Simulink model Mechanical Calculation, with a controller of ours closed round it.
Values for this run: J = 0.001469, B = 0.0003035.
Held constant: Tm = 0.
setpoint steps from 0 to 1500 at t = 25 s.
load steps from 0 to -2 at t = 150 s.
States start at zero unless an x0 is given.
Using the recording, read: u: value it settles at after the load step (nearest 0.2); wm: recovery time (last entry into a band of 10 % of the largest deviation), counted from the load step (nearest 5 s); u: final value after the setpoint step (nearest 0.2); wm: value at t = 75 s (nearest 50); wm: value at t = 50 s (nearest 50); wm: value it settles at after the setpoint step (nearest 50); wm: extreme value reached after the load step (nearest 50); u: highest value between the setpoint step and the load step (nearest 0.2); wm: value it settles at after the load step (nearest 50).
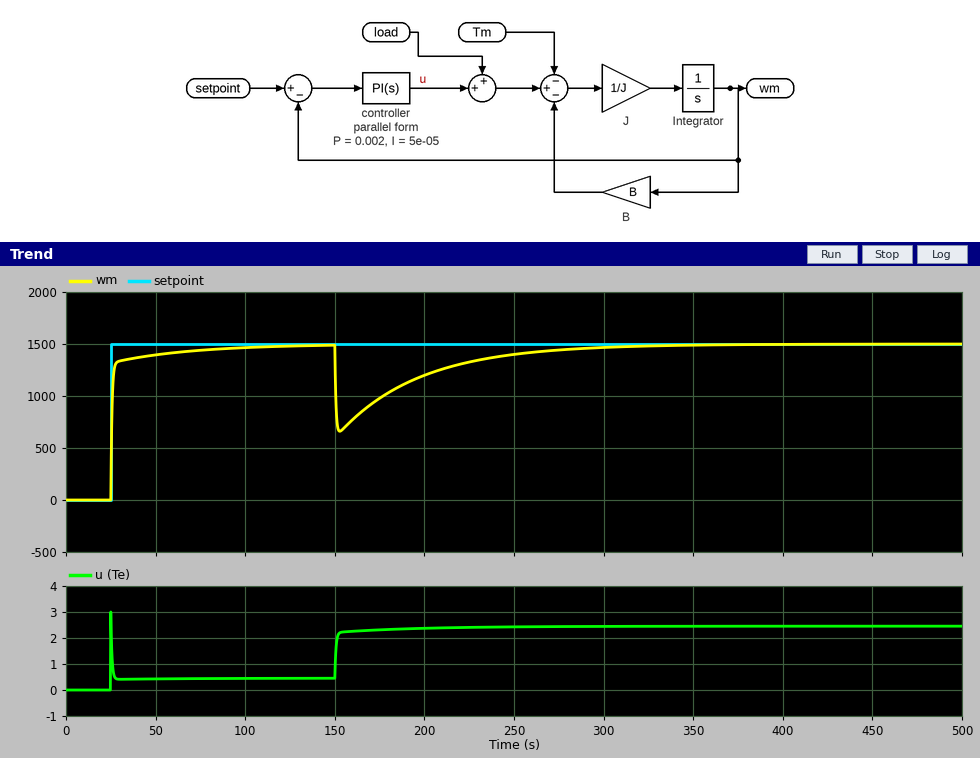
2.4
110 s
0.4
1450
1400
1500
650
3.0
1500
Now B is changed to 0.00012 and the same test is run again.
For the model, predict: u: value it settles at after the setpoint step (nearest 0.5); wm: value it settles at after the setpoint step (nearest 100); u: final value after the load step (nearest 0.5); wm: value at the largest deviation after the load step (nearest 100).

0.0
1500
2.0
600
